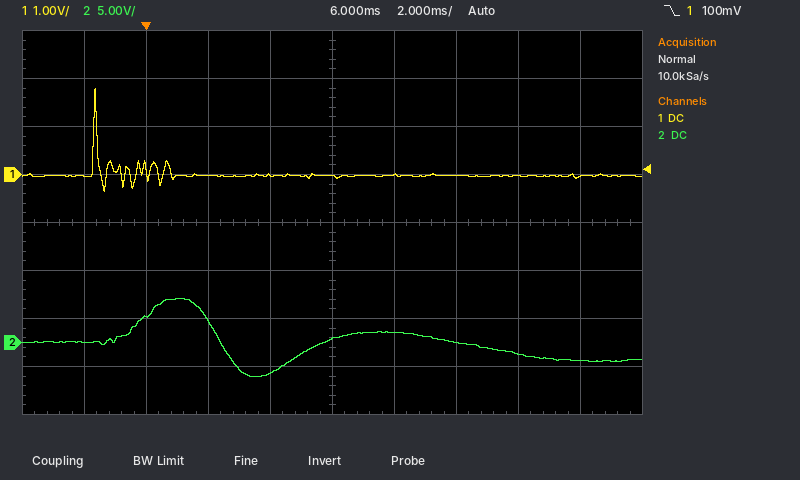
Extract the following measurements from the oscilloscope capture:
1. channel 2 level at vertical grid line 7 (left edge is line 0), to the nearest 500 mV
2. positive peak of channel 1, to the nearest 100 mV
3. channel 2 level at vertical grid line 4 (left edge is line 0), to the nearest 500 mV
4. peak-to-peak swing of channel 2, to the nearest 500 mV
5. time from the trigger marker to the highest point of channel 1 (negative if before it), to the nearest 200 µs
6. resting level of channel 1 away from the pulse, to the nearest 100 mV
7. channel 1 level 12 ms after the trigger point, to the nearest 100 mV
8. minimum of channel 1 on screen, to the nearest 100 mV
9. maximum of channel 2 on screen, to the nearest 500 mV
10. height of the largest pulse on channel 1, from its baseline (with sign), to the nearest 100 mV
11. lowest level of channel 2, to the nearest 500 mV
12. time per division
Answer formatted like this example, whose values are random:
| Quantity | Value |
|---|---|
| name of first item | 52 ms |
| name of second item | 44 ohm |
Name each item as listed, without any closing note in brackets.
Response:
| Quantity | Value |
|---|---|
| channel 2 level at vertical grid line 7 (left edge is line 0), to the nearest 500 mV | 0.0 V |
| positive peak of channel 1, to the nearest 100 mV | 1.8 V |
| channel 2 level at vertical grid line 4 (left edge is line 0), to the nearest 500 mV | -3.0 V |
| peak-to-peak swing of channel 2, to the nearest 500 mV | 8.0 V |
| time from the trigger marker to the highest point of channel 1 (negative if before it), to the nearest 200 µs | -1.6 ms |
| resting level of channel 1 away from the pulse, to the nearest 100 mV | 0.0 V |
| channel 1 level 12 ms after the trigger point, to the nearest 100 mV | 0.0 V |
| minimum of channel 1 on screen, to the nearest 100 mV | -400 mV |
| maximum of channel 2 on screen, to the nearest 500 mV | 4.5 V |
| height of the largest pulse on channel 1, from its baseline (with sign), to the nearest 100 mV | +1.8 V |
| lowest level of channel 2, to the nearest 500 mV | -3.5 V |
| time per division | 2 ms |
